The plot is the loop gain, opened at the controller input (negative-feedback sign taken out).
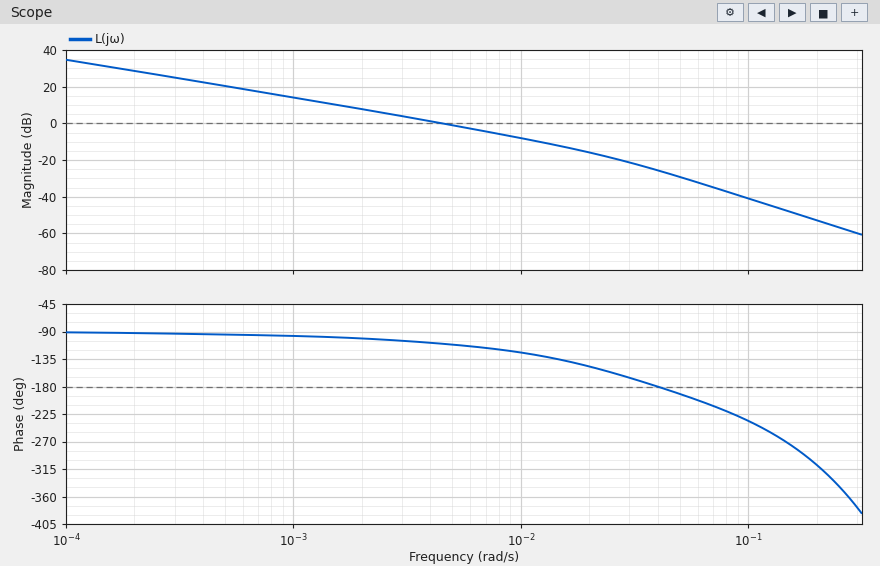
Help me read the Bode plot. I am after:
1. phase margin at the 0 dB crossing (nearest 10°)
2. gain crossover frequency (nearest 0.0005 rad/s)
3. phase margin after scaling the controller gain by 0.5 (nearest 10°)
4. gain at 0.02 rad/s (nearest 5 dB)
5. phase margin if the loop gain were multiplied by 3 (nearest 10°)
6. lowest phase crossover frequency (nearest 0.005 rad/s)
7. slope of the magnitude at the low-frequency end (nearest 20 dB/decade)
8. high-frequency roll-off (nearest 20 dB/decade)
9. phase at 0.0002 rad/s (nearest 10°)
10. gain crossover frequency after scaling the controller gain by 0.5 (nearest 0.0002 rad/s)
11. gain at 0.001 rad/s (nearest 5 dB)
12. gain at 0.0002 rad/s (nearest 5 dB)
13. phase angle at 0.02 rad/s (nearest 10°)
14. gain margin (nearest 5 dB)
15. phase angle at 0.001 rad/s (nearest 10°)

70°
0.0045 rad/s
80°
-15 dB
50°
0.040 rad/s
-20 dB/decade
-40 dB/decade
-90°
0.0024 rad/s
15 dB
30 dB
-150°
25 dB
-100°
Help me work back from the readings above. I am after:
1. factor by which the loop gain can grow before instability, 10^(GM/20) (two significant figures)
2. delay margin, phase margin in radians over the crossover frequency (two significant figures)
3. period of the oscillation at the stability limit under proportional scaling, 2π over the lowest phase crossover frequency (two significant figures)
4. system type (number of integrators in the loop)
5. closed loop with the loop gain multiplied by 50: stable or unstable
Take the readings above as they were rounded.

18
270 s
160 s
1
unstable
